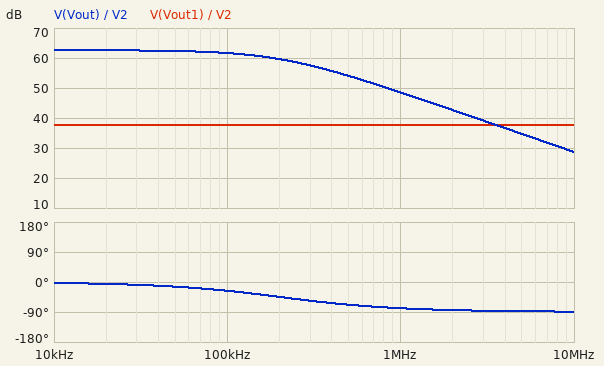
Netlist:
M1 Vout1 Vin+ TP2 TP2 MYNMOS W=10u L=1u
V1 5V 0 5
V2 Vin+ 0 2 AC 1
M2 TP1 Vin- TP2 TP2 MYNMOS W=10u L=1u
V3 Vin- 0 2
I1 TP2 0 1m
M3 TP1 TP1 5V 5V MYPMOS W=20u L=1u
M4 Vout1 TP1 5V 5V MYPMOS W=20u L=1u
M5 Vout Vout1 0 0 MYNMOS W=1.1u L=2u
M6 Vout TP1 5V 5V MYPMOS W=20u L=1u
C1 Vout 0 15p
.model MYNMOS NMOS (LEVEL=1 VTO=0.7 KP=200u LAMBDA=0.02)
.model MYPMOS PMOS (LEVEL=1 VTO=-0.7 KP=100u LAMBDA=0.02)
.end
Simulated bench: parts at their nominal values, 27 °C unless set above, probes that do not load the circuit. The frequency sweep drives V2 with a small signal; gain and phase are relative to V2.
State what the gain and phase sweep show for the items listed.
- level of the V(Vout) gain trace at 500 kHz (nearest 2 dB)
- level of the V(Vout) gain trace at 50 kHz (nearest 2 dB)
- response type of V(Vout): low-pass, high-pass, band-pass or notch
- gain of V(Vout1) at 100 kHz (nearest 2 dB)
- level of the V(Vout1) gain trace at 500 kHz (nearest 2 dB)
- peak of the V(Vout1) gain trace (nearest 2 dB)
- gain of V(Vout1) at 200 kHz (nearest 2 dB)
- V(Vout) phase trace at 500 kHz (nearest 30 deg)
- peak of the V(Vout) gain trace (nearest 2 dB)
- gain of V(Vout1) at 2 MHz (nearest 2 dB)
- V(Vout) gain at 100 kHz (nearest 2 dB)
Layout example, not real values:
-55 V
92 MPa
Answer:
54 dB
62 dB
low-pass
38 dB
38 dB
38 dB
38 dB
-60 deg
62 dB
38 dB
62 dB
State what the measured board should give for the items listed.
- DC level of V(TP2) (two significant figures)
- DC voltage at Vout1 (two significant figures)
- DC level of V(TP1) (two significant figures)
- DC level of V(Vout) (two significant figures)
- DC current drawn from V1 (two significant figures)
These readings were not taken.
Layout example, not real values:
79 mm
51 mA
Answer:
610 mV
3.6 V
3.6 V
3.8 V
1.5 mA
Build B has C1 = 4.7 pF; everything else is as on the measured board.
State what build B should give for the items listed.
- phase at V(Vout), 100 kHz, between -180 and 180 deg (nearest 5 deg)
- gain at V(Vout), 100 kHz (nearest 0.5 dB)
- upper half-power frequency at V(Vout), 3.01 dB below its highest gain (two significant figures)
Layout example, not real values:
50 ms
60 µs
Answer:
-10 deg
62.5 dB
640 kHz
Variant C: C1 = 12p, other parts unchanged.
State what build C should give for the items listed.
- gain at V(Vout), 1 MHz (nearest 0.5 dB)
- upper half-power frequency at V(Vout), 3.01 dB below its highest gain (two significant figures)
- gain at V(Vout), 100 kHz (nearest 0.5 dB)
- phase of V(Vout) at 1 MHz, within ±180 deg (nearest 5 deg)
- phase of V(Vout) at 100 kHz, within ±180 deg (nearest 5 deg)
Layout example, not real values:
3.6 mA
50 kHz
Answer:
50.5 dB
250 kHz
62.0 dB
-75 deg
-20 deg
